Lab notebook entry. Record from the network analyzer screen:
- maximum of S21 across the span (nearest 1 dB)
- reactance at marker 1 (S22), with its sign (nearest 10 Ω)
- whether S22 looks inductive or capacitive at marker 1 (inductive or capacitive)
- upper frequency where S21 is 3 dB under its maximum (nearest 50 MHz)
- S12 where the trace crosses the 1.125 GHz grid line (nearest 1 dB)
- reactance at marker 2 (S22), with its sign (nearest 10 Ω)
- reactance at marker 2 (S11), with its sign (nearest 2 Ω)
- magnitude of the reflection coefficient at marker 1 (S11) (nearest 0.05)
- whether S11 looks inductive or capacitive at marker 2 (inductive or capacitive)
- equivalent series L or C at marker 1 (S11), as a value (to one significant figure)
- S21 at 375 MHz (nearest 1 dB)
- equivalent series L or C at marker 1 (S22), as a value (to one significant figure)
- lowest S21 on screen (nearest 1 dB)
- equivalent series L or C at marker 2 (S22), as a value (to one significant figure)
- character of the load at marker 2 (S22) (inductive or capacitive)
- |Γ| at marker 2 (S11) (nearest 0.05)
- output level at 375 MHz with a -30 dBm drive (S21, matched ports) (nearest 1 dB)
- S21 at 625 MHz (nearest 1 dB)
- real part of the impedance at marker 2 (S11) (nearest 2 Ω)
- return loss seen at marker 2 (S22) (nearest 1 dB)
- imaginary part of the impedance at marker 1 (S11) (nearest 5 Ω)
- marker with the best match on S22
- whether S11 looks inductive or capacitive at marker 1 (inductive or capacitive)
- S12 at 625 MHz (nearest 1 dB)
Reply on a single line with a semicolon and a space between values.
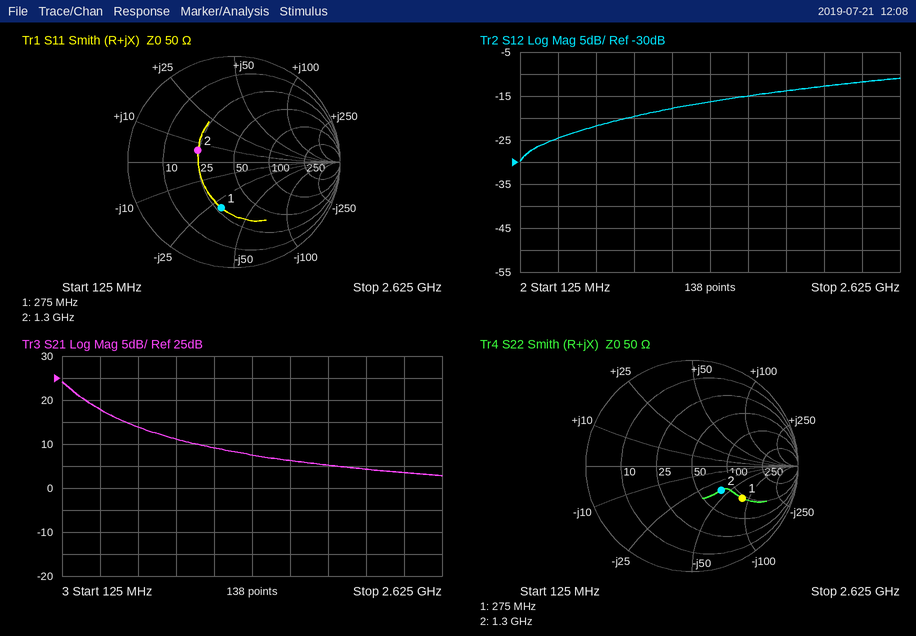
24 dB; -80 Ω; capacitive; 250 MHz; -18 dB; -40 Ω; +6 Ω; 0.45; inductive; 20 pF; 18 dB; 7 pF; 3 dB; 3 pF; capacitive; 0.35; -12 dBm; 14 dB; 24 Ω; 9 dB; -30 Ω; marker 2; capacitive; -22 dB
